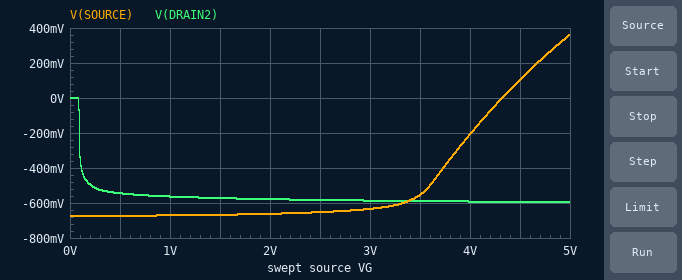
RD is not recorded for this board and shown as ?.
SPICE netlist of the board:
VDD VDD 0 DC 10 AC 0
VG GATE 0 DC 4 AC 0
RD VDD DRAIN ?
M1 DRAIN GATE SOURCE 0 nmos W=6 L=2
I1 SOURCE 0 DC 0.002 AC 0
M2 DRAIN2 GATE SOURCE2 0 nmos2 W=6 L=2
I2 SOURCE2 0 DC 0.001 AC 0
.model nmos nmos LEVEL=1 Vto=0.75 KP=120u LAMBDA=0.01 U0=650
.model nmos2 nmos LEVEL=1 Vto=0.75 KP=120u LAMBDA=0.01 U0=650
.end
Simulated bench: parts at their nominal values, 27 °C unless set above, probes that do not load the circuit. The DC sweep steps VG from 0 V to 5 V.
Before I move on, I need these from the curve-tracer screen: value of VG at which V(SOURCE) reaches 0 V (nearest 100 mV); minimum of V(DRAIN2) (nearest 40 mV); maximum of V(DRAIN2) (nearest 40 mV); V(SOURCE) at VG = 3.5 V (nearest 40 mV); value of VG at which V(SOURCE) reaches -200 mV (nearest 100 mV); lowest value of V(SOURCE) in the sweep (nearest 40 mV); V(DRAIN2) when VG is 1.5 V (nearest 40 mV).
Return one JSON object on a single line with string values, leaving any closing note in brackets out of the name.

{"value of VG at which V(SOURCE) reaches 0 V": "4.3 V", "minimum of V(DRAIN2)": "-600 mV", "maximum of V(DRAIN2)": "0 V", "V(SOURCE) at VG = 3.5 V": "-560 mV", "value of VG at which V(SOURCE) reaches -200 mV": "4.0 V", "lowest value of V(SOURCE) in the sweep": "-680 mV", "V(DRAIN2) when VG is 1.5 V": "-560 mV"}
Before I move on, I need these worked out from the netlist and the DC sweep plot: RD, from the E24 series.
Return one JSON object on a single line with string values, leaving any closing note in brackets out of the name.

{"RD, from the E24 series": "3.9 kΩ"}
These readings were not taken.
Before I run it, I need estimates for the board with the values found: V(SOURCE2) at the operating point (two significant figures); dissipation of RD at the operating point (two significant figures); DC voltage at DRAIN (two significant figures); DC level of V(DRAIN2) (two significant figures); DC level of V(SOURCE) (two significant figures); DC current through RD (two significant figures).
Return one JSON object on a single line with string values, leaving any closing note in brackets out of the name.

{"V(SOURCE2) at the operating point": "-650 mV", "dissipation of RD at the operating point": "16 mW", "DC voltage at DRAIN": "2.2 V", "DC level of V(DRAIN2)": "-590 mV", "DC level of V(SOURCE)": "-210 mV", "DC current through RD": "2.0 mA"}
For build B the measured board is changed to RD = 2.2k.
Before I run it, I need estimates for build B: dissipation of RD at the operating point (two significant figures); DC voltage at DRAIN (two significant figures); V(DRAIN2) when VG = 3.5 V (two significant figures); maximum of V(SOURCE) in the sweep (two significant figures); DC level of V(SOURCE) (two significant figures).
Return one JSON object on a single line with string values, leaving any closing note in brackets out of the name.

{"dissipation of RD at the operating point": "8.8 mW", "DC voltage at DRAIN": "5.6 V", "V(DRAIN2) when VG = 3.5 V": "-590 mV", "maximum of V(SOURCE) in the sweep": "990 mV", "DC level of V(SOURCE)": "6.2 mV"}
